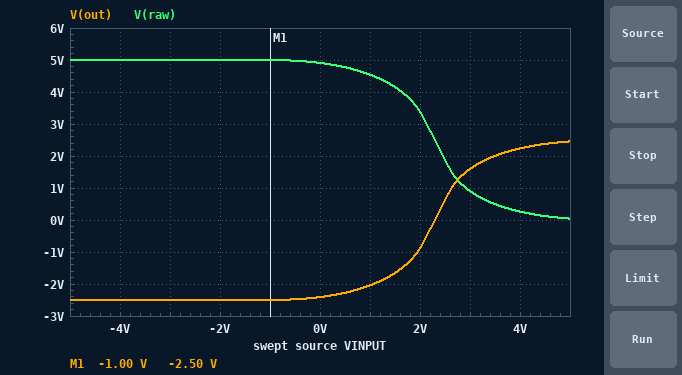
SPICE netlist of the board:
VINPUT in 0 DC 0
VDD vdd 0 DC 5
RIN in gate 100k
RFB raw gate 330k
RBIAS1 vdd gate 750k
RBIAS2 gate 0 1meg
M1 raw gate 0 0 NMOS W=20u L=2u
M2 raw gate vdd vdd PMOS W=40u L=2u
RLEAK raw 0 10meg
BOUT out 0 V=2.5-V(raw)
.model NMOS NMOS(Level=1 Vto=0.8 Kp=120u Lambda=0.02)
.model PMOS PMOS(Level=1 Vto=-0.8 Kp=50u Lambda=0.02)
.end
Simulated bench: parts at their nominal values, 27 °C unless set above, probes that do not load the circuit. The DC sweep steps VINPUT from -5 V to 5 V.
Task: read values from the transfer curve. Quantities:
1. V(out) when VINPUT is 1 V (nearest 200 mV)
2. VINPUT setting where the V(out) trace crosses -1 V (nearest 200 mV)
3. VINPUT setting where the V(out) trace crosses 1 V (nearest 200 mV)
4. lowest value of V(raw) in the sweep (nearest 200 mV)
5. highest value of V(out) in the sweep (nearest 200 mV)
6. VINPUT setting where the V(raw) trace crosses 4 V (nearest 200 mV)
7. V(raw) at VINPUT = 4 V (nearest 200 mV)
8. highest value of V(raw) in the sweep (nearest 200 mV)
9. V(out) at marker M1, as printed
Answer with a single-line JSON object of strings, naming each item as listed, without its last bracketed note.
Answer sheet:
{"V(out) when VINPUT is 1 V": "-2.0 V", "VINPUT setting where the V(out) trace crosses -1 V": "2.0 V", "VINPUT setting where the V(out) trace crosses 1 V": "2.6 V", "lowest value of V(raw) in the sweep": "0 V", "highest value of V(out) in the sweep": "2.4 V", "VINPUT setting where the V(raw) trace crosses 4 V": "1.6 V", "V(raw) at VINPUT = 4 V": "200 mV", "highest value of V(raw) in the sweep": "5.0 V", "V(out) at marker M1, as printed": "-2.50 V"}
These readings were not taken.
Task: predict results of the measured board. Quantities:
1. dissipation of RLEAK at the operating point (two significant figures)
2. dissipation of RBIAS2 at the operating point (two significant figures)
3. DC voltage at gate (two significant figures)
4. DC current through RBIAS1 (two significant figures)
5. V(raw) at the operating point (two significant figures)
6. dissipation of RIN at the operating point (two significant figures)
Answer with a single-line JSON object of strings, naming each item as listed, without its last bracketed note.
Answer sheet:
{"dissipation of RLEAK at the operating point": "2.4 µW", "dissipation of RBIAS2 at the operating point": "2.0 µW", "DC voltage at gate": "1.4 V", "DC current through RBIAS1": "4.8 µA", "V(raw) at the operating point": "4.9 V", "dissipation of RIN at the operating point": "20 µW"}
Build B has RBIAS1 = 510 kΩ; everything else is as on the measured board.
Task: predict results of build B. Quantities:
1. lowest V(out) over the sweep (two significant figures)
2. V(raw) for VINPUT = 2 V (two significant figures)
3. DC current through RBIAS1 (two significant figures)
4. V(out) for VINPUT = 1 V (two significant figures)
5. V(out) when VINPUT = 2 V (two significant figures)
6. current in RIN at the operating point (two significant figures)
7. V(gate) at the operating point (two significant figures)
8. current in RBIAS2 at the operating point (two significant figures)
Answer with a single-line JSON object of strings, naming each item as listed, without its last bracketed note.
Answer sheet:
{"lowest V(out) over the sweep": "-2.5 V", "V(raw) for VINPUT = 2 V": "2.9 V", "DC current through RBIAS1": "6.8 µA", "V(out) for VINPUT = 1 V": "-1.9 V", "V(out) when VINPUT = 2 V": "-410 mV", "current in RIN at the operating point": "15 µA", "V(gate) at the operating point": "1.5 V", "current in RBIAS2 at the operating point": "1.5 µA"}
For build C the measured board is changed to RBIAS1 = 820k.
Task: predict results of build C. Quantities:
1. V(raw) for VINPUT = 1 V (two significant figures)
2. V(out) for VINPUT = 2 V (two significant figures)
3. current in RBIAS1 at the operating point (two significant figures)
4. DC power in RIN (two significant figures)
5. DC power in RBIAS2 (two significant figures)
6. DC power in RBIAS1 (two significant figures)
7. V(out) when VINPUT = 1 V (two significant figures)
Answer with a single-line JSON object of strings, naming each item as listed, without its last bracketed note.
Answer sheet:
{"V(raw) for VINPUT = 1 V": "4.6 V", "V(out) for VINPUT = 2 V": "-950 mV", "current in RBIAS1 at the operating point": "4.4 µA", "DC power in RIN": "19 µW", "DC power in RBIAS2": "1.9 µW", "DC power in RBIAS1": "16 µW", "V(out) when VINPUT = 1 V": "-2.1 V"}
